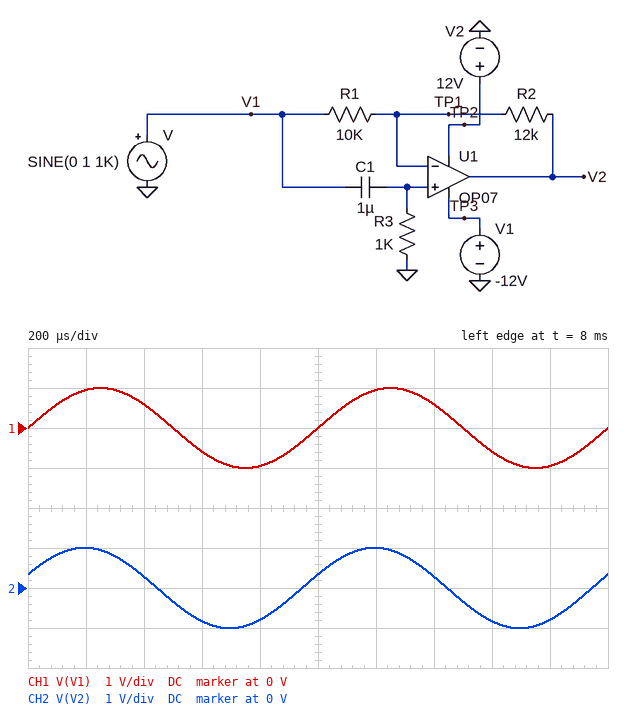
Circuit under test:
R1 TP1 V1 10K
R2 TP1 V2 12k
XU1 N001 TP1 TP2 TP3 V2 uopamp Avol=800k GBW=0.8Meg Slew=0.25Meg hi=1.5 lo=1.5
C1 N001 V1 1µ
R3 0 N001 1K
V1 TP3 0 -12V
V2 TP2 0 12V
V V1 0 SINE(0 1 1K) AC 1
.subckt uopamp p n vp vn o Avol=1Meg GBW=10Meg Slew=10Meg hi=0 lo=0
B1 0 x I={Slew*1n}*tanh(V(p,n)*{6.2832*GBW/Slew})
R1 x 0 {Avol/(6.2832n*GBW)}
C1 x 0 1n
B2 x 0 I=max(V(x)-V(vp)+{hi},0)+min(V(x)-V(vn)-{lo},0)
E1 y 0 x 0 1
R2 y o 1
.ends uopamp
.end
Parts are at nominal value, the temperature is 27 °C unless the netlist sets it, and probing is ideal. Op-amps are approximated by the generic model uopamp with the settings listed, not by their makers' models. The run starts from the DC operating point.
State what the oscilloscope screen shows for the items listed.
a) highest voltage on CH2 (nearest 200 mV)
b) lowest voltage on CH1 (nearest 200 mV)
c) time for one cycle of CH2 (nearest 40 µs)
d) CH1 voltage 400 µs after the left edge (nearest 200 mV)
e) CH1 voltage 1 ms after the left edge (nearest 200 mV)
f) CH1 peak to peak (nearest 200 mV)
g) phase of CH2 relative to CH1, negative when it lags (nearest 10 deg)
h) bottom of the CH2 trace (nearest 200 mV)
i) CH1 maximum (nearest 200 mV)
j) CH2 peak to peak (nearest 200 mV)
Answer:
1.0 V
-1.0 V
1.00 ms
600 mV
0 V
2.0 V
20 deg
-1.0 V
1.0 V
2.0 V
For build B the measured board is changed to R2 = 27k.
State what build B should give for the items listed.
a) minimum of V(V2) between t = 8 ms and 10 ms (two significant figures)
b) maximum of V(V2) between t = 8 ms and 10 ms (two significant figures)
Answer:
-1.1 V
1.1 V
